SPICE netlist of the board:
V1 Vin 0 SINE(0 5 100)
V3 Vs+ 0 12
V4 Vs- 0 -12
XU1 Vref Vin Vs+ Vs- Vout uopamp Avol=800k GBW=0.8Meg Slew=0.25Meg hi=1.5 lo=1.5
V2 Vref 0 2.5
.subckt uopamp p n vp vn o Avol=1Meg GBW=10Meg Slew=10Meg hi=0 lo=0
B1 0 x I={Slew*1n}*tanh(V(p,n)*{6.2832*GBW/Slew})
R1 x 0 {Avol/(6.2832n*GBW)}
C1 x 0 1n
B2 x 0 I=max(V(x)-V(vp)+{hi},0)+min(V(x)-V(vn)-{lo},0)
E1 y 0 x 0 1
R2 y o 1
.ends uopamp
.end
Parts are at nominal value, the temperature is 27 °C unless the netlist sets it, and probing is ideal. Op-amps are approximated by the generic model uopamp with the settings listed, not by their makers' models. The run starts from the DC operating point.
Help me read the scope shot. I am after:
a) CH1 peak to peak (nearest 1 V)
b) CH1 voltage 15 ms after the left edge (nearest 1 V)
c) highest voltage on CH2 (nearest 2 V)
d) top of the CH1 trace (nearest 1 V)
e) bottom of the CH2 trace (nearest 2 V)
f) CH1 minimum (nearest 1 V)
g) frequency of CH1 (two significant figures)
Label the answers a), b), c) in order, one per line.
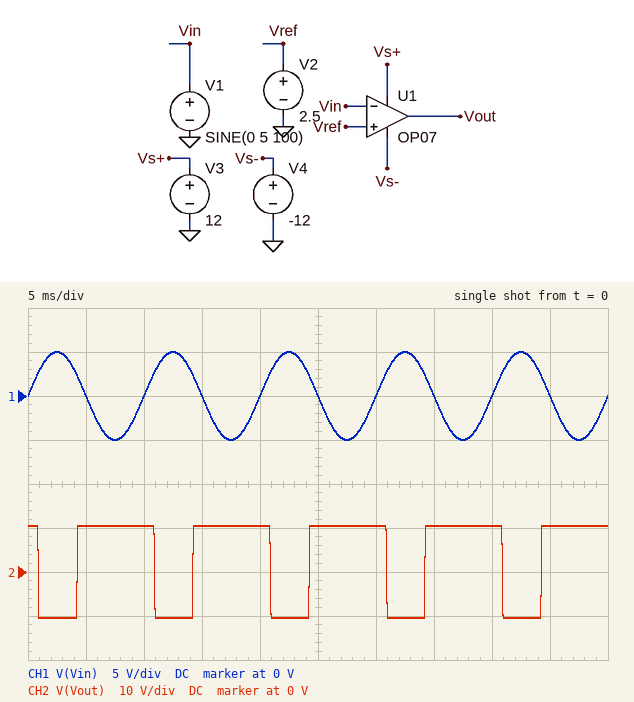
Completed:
a) 10 V
b) 0 V
c) 10 V
d) 5 V
e) -10 V
f) -5 V
g) 100 Hz
